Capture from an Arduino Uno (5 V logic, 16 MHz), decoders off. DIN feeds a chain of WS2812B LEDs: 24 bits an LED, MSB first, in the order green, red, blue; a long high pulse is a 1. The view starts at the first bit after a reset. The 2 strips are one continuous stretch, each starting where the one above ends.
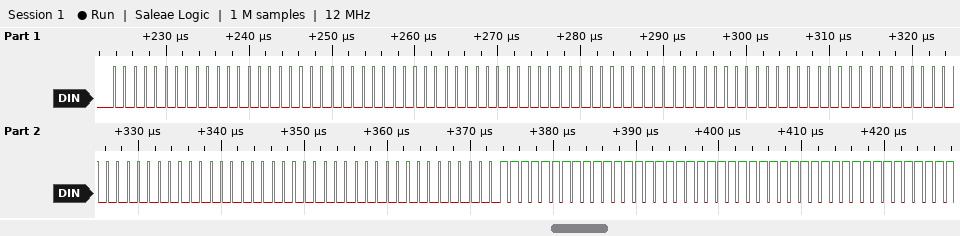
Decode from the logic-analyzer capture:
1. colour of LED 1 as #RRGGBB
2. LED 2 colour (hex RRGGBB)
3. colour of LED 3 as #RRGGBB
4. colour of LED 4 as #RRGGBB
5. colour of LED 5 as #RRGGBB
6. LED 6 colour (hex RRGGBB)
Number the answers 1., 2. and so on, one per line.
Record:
1. #000000
2. #000000
3. #000000
4. #000000
5. #000000
6. #FFFFFF
